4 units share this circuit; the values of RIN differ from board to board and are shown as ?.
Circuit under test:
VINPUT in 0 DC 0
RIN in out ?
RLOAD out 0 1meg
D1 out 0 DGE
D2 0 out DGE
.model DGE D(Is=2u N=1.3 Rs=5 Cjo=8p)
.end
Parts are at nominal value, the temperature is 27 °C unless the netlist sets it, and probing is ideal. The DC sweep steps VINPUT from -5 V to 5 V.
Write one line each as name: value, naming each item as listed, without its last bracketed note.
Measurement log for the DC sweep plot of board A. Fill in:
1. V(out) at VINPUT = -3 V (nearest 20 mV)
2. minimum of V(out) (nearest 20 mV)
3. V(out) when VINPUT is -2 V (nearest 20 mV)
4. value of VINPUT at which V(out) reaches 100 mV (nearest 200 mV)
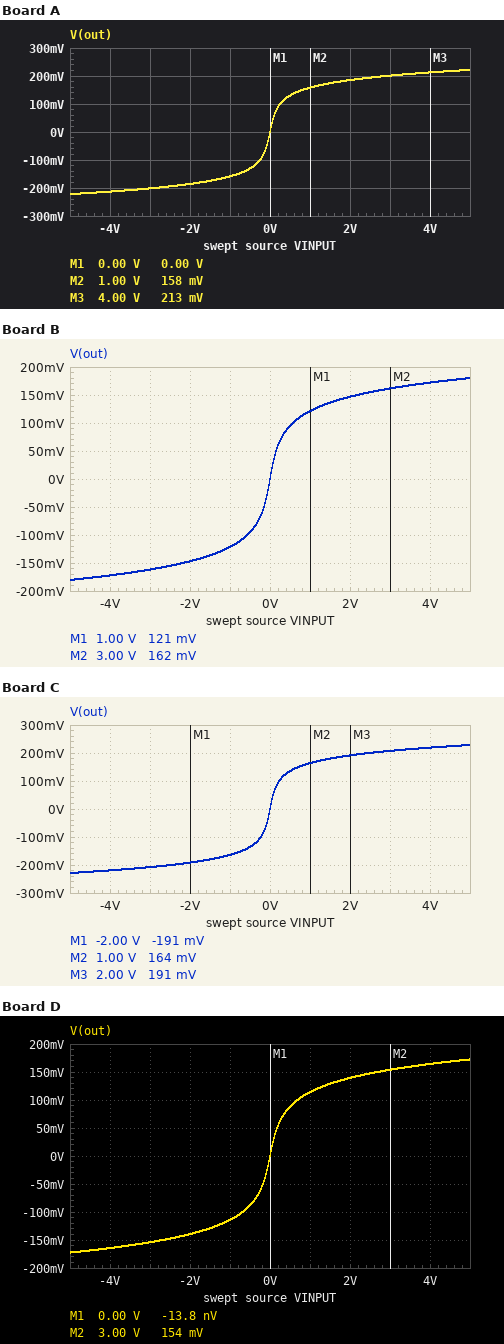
V(out) at VINPUT = -3 V: -200 mV
minimum of V(out): -220 mV
V(out) when VINPUT is -2 V: -180 mV
value of VINPUT at which V(out) reaches 100 mV: 200 mV
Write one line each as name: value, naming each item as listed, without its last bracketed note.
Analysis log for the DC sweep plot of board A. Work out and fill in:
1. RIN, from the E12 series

RIN, from the E12 series: 3.9 kΩ
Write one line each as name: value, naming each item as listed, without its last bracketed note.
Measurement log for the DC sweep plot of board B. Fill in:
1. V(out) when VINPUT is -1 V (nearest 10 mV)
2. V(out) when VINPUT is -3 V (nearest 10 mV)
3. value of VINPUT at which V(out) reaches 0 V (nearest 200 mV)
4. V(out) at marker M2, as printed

V(out) when VINPUT is -1 V: -120 mV
V(out) when VINPUT is -3 V: -160 mV
value of VINPUT at which V(out) reaches 0 V: 0 V
V(out) at marker M2, as printed: 162 mV
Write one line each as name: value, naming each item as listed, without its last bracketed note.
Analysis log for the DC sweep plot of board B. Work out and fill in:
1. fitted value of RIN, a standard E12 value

fitted value of RIN, a standard E12 value: 12 kΩ
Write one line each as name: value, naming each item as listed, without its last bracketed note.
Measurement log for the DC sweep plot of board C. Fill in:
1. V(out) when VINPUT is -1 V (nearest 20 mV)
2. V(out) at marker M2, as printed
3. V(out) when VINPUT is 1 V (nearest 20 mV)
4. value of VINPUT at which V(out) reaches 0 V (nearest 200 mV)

V(out) when VINPUT is -1 V: -160 mV
V(out) at marker M2, as printed: 164 mV
V(out) when VINPUT is 1 V: 160 mV
value of VINPUT at which V(out) reaches 0 V: 0 V
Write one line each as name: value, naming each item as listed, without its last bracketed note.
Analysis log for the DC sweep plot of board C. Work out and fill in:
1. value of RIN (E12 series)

value of RIN: 3.3 kΩ
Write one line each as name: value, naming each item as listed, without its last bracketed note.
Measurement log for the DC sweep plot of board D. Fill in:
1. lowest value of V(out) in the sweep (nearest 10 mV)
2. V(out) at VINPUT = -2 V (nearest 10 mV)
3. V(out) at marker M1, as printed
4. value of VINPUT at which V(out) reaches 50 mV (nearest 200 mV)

lowest value of V(out) in the sweep: -170 mV
V(out) at VINPUT = -2 V: -140 mV
V(out) at marker M1, as printed: -13.8 nV
value of VINPUT at which V(out) reaches 50 mV: 200 mV
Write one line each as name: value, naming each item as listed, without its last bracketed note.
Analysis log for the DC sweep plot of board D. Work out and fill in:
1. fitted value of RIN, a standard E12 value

fitted value of RIN, a standard E12 value: 15 kΩ
